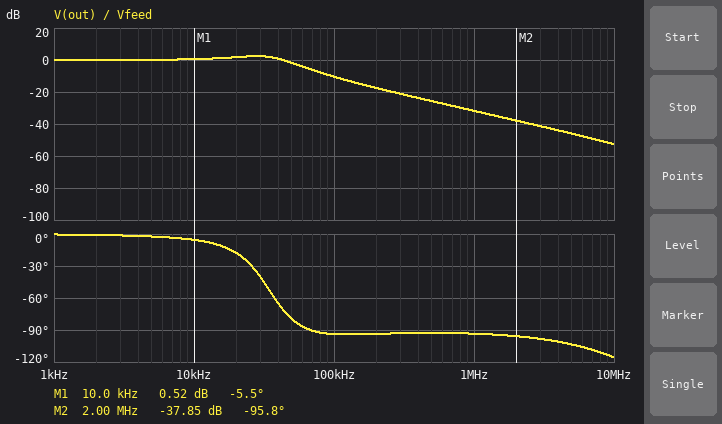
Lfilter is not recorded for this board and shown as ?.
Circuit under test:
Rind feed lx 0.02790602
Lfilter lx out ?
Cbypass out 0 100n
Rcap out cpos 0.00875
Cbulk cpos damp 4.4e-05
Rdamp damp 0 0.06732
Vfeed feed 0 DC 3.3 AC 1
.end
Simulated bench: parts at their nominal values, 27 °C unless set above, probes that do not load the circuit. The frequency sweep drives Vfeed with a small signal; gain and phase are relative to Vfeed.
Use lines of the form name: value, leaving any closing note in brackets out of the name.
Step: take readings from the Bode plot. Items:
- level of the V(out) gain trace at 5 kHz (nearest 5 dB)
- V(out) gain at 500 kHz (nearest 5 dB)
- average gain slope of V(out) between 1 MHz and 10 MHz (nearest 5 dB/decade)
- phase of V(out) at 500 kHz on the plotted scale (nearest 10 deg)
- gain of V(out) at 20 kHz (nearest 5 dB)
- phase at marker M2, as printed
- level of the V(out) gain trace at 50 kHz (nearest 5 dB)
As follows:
level of the V(out) gain trace at 5 kHz: 0 dB
V(out) gain at 500 kHz: -25 dB
average gain slope of V(out) between 1 MHz and 10 MHz: -20 dB/decade
phase of V(out) at 500 kHz on the plotted scale: -90 deg
gain of V(out) at 20 kHz: 0 dB
phase at marker M2, as printed: -95.8 deg
level of the V(out) gain trace at 50 kHz: 0 dB
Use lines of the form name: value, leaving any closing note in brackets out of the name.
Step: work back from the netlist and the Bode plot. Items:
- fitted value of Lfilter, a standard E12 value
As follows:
fitted value of Lfilter, a standard E12 value: 470 nH
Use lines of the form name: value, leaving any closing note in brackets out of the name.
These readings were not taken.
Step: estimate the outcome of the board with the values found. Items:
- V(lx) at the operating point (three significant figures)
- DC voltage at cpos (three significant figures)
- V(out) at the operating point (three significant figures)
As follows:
V(lx) at the operating point: 3.30 V
DC voltage at cpos: 3.30 V
V(out) at the operating point: 3.30 V
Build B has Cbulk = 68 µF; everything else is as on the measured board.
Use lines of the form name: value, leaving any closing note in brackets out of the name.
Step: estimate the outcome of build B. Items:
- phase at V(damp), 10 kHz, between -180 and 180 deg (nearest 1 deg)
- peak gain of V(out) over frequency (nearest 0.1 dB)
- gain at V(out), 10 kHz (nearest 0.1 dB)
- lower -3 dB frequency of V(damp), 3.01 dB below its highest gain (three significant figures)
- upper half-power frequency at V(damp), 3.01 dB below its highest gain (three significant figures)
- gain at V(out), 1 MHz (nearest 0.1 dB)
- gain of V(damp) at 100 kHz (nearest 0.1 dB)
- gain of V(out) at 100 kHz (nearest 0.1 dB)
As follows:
phase at V(damp), 10 kHz, between -180 and 180 deg: 63 deg
peak gain of V(out) over frequency: 1.4 dB
gain at V(out), 10 kHz: 0.6 dB
lower -3 dB frequency of V(damp), 3.01 dB below its highest gain: 15.6 kHz
upper half-power frequency at V(damp), 3.01 dB below its highest gain: 50.8 kHz
gain at V(out), 1 MHz: -31.8 dB
gain of V(damp) at 100 kHz: -12.7 dB
gain of V(out) at 100 kHz: -11.3 dB
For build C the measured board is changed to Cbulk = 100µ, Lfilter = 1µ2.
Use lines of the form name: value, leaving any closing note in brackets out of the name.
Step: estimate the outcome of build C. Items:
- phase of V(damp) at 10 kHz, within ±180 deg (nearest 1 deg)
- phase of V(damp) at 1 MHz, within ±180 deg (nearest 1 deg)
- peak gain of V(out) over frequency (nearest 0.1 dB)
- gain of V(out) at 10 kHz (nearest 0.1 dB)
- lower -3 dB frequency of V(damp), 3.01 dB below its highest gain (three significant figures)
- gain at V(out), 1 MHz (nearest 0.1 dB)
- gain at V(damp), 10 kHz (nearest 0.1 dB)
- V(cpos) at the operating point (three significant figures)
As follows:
phase of V(damp) at 10 kHz, within ±180 deg: 39 deg
phase of V(damp) at 1 MHz, within ±180 deg: -92 deg
peak gain of V(out) over frequency: 2.7 dB
gain of V(out) at 10 kHz: 2.4 dB
lower -3 dB frequency of V(damp), 3.01 dB below its highest gain: 9.19 kHz
gain at V(out), 1 MHz: -39.9 dB
gain at V(damp), 10 kHz: -5.9 dB
V(cpos) at the operating point: 3.30 V
